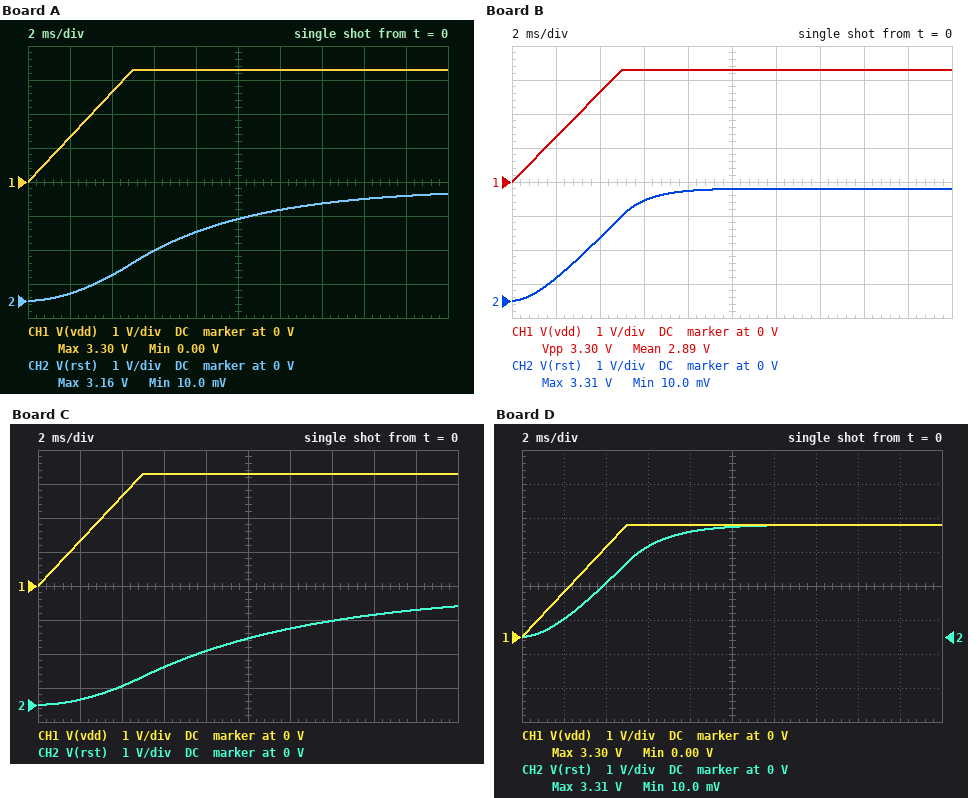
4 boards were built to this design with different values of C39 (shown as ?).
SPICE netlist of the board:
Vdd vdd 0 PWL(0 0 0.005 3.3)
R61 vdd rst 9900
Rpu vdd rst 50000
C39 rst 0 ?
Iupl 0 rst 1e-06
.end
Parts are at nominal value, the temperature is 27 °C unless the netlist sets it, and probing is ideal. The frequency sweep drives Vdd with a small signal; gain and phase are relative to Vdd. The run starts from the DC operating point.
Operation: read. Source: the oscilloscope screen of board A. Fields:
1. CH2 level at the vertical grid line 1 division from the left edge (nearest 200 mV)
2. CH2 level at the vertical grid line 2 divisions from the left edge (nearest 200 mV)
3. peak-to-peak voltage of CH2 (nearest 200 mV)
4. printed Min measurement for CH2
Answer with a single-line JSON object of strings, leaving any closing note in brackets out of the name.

{"CH2 level at the vertical grid line 1 division from the left edge": "200 mV", "CH2 level at the vertical grid line 2 divisions from the left edge": "800 mV", "peak-to-peak voltage of CH2": "3.2 V", "printed Min measurement for CH2": "10.0 mV"}
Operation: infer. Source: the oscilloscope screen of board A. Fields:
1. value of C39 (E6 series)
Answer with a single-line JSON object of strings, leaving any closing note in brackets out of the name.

{"value of C39": "680 nF"}
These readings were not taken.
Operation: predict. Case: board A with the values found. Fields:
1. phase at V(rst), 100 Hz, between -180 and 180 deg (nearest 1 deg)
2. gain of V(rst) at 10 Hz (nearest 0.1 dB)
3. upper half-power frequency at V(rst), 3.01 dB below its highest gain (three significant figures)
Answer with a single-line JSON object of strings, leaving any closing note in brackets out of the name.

{"phase at V(rst), 100 Hz, between -180 and 180 deg": "-74 deg", "gain of V(rst) at 10 Hz": "-0.5 dB", "upper half-power frequency at V(rst), 3.01 dB below its highest gain": "28.3 Hz"}
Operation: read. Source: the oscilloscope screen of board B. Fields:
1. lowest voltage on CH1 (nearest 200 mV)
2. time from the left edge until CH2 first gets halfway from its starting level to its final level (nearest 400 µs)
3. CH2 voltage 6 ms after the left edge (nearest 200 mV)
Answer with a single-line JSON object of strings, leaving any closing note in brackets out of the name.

{"lowest voltage on CH1": "0 V", "time from the left edge until CH2 first gets halfway from its starting level to its final level": "3.6 ms", "CH2 voltage 6 ms after the left edge": "3.0 V"}
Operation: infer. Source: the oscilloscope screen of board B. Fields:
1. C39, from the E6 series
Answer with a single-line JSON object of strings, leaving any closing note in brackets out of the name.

{"C39, from the E6 series": "150 nF"}
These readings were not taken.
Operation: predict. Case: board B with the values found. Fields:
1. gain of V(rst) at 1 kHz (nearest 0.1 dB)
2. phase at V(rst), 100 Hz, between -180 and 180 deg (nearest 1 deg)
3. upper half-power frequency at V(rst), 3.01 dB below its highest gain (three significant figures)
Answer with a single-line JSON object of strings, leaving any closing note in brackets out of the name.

{"gain of V(rst) at 1 kHz": "-17.9 dB", "phase at V(rst), 100 Hz, between -180 and 180 deg": "-38 deg", "upper half-power frequency at V(rst), 3.01 dB below its highest gain": "128 Hz"}
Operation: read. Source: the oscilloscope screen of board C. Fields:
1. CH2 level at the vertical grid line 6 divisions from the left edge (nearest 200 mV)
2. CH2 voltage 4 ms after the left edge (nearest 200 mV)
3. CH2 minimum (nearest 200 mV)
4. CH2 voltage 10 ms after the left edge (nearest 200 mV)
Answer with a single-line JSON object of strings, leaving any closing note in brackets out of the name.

{"CH2 level at the vertical grid line 6 divisions from the left edge": "2.2 V", "CH2 voltage 4 ms after the left edge": "600 mV", "CH2 minimum": "0 V", "CH2 voltage 10 ms after the left edge": "2.0 V"}
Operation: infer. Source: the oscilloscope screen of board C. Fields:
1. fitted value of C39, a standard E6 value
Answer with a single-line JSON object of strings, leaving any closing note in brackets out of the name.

{"fitted value of C39, a standard E6 value": "1 µF"}
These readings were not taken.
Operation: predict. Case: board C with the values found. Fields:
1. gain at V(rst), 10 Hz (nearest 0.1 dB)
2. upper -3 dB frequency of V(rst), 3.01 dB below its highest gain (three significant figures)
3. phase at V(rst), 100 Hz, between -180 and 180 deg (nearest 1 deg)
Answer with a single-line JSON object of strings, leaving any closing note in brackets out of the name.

{"gain at V(rst), 10 Hz": "-1.0 dB", "upper -3 dB frequency of V(rst), 3.01 dB below its highest gain": "19.3 Hz", "phase at V(rst), 100 Hz, between -180 and 180 deg": "-79 deg"}
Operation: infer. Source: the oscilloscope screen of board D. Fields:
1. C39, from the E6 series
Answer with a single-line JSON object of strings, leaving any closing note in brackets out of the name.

{"C39, from the E6 series": "220 nF"}
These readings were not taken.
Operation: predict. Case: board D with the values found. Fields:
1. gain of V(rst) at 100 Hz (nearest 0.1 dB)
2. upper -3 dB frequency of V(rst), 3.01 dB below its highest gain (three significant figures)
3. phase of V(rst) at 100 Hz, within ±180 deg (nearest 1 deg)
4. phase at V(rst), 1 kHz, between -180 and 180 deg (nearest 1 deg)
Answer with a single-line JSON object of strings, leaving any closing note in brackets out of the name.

{"gain of V(rst) at 100 Hz": "-3.6 dB", "upper -3 dB frequency of V(rst), 3.01 dB below its highest gain": "87.5 Hz", "phase of V(rst) at 100 Hz, within ±180 deg": "-49 deg", "phase at V(rst), 1 kHz, between -180 and 180 deg": "-85 deg"}
